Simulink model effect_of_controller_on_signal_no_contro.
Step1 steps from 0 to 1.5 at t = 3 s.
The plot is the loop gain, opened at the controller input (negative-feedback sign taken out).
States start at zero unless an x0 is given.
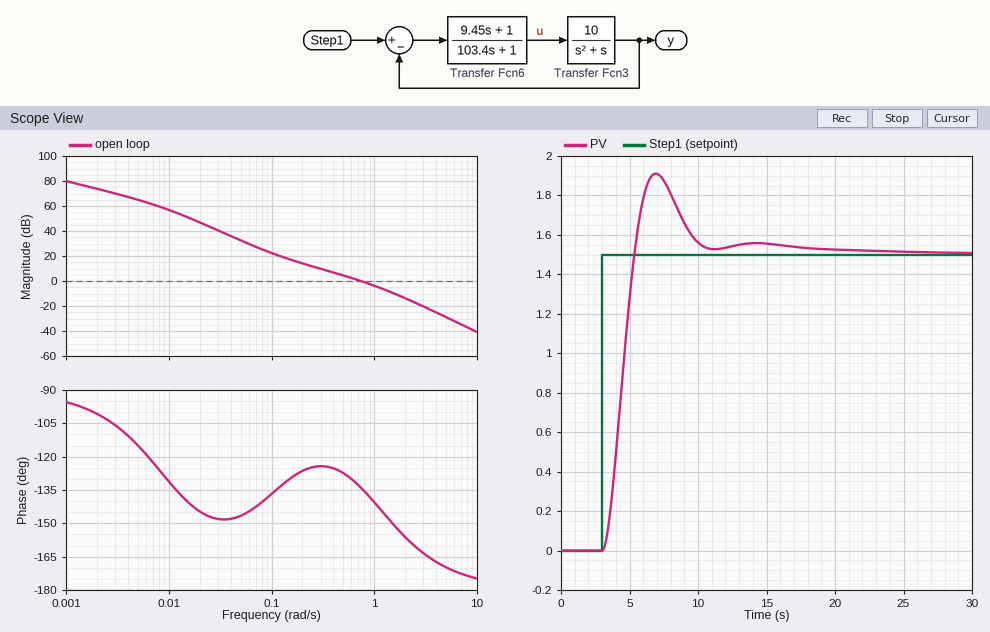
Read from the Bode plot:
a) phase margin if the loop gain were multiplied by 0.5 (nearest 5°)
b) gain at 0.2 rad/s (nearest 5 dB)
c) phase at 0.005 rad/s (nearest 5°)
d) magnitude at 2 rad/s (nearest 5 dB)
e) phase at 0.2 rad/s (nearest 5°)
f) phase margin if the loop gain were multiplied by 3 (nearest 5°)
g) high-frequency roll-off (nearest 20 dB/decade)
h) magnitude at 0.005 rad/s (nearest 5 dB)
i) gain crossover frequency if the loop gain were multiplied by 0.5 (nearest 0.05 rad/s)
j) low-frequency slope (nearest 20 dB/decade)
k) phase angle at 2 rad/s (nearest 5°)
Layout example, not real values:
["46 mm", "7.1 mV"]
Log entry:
["55°", "15 dB", "-115°", "-15 dB", "-125°", "30°", "-40 dB/decade", "65 dB", "0.45 rad/s", "-20 dB/decade", "-155°"]
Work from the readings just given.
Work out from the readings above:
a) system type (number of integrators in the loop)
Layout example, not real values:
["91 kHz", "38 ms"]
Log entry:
["1"]
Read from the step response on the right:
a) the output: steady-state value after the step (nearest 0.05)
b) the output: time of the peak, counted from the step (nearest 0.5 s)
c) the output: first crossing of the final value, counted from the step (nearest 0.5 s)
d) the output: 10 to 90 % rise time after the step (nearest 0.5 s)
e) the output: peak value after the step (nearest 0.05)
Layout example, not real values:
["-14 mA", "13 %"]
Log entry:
["1.50", "4.0 s", "2.5 s", "1.5 s", "1.90"]
